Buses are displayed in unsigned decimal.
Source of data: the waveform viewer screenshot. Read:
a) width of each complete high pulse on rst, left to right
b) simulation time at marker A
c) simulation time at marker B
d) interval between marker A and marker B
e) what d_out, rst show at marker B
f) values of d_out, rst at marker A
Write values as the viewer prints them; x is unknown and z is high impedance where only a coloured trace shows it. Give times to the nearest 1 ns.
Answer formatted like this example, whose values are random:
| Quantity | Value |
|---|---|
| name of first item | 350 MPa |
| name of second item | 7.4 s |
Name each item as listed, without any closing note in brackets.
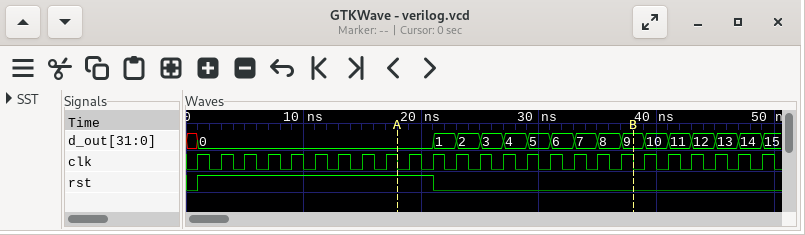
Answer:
| Quantity | Value |
|---|---|
| width of each complete high pulse on rst, left to right | 20 ns |
| simulation time at marker A | 18 ns |
| simulation time at marker B | 38 ns |
| interval between marker A and marker B | 20 ns |
| what d_out, rst show at marker B | d_out=9, rst=0 |
| values of d_out, rst at marker A | d_out=0, rst=1 |
